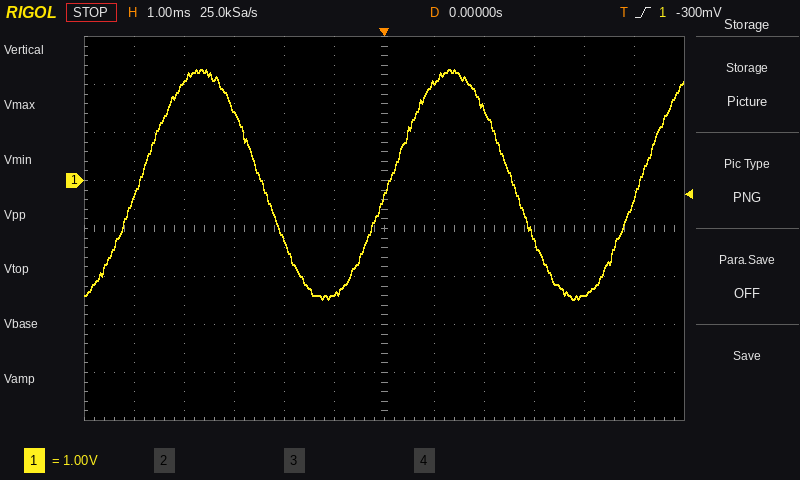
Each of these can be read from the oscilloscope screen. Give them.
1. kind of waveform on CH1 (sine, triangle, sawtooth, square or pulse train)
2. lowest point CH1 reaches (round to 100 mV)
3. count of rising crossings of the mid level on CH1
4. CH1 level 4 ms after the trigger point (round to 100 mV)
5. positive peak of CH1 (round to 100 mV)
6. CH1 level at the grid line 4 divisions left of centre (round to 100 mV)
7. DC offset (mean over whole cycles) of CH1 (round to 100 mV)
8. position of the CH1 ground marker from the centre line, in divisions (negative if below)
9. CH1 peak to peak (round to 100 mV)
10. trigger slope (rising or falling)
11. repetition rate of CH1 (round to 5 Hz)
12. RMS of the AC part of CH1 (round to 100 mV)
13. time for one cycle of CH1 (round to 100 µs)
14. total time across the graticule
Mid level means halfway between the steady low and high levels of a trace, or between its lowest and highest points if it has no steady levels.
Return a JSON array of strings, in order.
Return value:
["sine", "-2.5 V", "3", "-2.4 V", "2.3 V", "2.1 V", "-100 mV", "+1.0 div", "4.8 V", "rising", "200 Hz", "1.7 V", "5.0 ms", "12 ms"]
